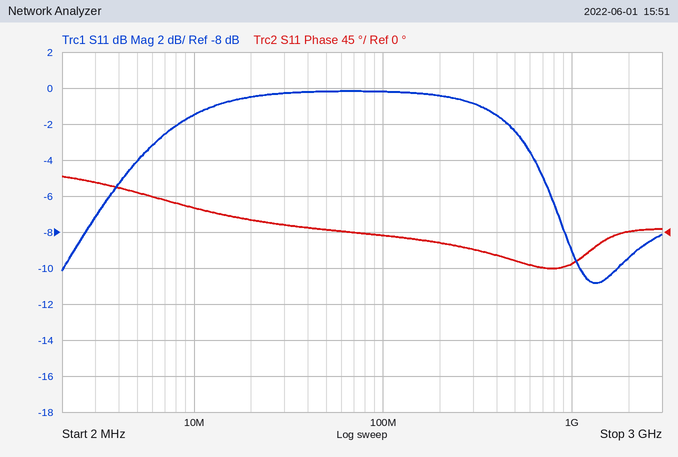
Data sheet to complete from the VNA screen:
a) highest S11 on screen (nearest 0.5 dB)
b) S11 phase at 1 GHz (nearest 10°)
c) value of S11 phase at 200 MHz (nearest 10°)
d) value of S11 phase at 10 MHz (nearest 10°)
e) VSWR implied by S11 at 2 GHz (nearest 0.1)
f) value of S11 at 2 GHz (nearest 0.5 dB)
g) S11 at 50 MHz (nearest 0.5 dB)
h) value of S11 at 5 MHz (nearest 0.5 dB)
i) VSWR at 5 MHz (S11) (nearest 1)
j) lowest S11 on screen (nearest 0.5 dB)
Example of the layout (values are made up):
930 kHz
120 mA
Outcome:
0.0 dB
-40°
-10°
30°
2.0
-9.5 dB
0.0 dB
-4.0 dB
4
-11.0 dB
